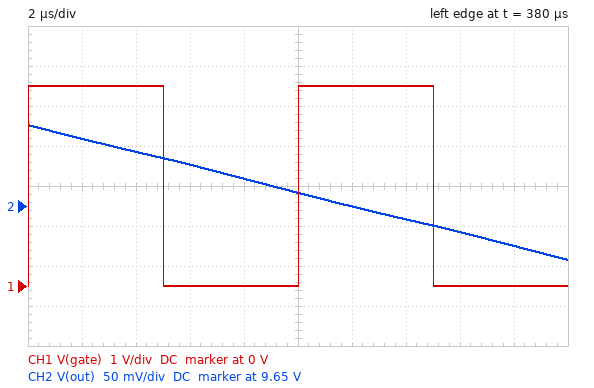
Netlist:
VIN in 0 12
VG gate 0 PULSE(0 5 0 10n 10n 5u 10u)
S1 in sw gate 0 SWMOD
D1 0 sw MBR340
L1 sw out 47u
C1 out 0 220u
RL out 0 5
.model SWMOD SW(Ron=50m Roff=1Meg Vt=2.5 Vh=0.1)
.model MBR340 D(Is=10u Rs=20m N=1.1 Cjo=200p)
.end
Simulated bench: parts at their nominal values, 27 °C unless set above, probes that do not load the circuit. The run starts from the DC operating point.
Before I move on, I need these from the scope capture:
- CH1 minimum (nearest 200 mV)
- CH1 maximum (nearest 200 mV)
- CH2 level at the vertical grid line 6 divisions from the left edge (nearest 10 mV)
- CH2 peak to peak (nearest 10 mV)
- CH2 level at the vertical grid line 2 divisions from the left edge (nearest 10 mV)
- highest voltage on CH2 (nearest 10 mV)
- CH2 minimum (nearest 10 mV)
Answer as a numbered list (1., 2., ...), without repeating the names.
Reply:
1. 0 V
2. 5.0 V
3. 9.65 V
4. 170 mV
5. 9.72 V
6. 9.75 V
7. 9.58 V
